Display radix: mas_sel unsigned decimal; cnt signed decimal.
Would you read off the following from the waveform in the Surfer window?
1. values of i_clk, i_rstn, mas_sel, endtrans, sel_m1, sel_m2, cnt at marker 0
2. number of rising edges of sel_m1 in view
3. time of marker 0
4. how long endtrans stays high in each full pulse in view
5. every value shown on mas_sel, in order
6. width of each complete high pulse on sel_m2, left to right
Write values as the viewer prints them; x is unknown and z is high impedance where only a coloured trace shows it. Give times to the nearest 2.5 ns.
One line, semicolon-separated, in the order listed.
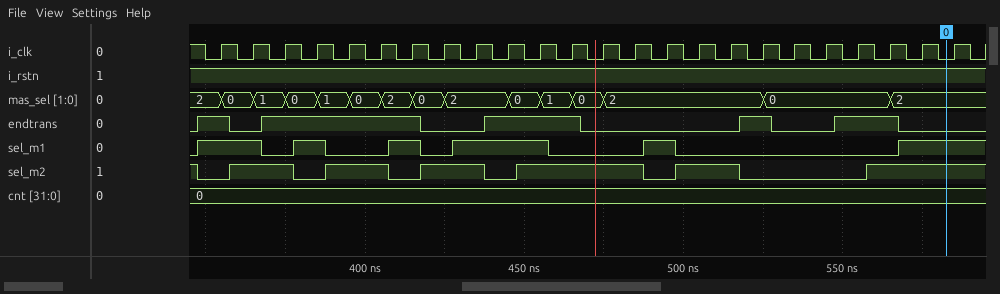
i_clk=0, i_rstn=1, mas_sel=2, endtrans=0, sel_m1=1, sel_m2=1, cnt=0; 6; 582.5 ns; 10 ns, 50 ns, 30 ns, 10 ns, 20 ns; 2, 0, 1, 0, 1, 0, 2, 0, 2, 0, 1, 0, 2, 0, 2; 20 ns, 20 ns, 20 ns, 40 ns, 20 ns
